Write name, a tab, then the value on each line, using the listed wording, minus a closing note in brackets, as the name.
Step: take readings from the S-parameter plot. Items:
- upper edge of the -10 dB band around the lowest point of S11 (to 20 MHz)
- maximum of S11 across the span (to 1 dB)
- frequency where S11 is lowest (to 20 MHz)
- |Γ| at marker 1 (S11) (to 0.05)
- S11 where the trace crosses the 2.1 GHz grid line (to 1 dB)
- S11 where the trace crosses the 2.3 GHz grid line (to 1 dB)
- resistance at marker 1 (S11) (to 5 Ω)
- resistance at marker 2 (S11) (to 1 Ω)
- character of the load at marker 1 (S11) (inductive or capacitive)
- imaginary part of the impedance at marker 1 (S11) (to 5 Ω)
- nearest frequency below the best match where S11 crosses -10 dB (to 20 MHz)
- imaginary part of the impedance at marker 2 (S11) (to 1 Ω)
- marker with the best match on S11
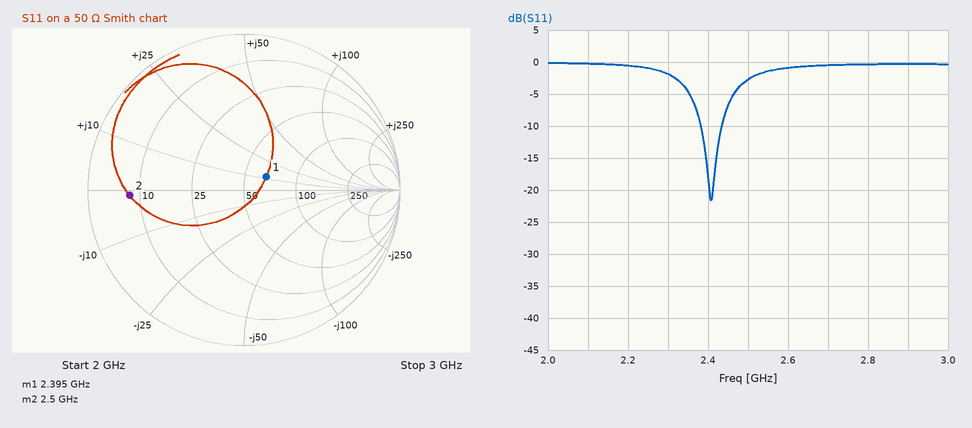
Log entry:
upper edge of the -10 dB band around the lowest point of S11	2.44 GHz
maximum of S11 across the span	0 dB
frequency where S11 is lowest	2.40 GHz
|Γ| at marker 1 (S11)	0.15
S11 where the trace crosses the 2.1 GHz grid line	0 dB
S11 where the trace crosses the 2.3 GHz grid line	-2 dB
resistance at marker 1 (S11)	65 Ω
resistance at marker 2 (S11)	8 Ω
character of the load at marker 1 (S11)	inductive
imaginary part of the impedance at marker 1 (S11)	+10 Ω
nearest frequency below the best match where S11 crosses -10 dB	2.38 GHz
imaginary part of the impedance at marker 2 (S11)	-1 Ω
marker with the best match on S11	marker 1
